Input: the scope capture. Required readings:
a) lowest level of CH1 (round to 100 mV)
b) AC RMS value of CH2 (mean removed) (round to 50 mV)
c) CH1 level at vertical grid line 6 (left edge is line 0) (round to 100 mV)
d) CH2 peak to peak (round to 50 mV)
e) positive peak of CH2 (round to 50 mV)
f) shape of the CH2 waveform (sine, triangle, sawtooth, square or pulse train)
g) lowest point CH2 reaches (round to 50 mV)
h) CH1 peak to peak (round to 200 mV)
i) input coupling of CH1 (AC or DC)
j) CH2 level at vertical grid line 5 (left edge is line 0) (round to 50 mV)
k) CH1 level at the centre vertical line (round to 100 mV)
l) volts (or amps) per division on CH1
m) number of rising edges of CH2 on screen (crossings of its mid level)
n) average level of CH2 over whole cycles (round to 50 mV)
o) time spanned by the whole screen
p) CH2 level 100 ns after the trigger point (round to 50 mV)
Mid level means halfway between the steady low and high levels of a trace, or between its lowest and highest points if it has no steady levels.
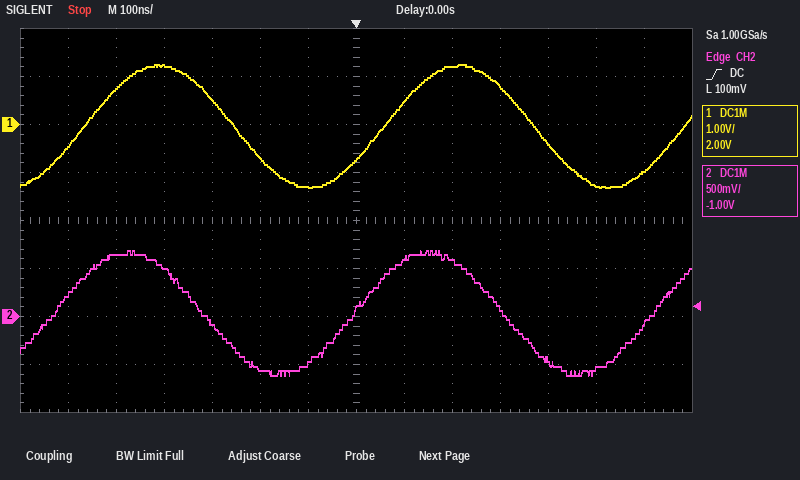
-1.3 V
450 mV
-1.3 V
1.30 V
700 mV
sine
-600 mV
2.6 V
DC
-550 mV
-700 mV
1 V
3
50 mV
1.4 µs
600 mV
